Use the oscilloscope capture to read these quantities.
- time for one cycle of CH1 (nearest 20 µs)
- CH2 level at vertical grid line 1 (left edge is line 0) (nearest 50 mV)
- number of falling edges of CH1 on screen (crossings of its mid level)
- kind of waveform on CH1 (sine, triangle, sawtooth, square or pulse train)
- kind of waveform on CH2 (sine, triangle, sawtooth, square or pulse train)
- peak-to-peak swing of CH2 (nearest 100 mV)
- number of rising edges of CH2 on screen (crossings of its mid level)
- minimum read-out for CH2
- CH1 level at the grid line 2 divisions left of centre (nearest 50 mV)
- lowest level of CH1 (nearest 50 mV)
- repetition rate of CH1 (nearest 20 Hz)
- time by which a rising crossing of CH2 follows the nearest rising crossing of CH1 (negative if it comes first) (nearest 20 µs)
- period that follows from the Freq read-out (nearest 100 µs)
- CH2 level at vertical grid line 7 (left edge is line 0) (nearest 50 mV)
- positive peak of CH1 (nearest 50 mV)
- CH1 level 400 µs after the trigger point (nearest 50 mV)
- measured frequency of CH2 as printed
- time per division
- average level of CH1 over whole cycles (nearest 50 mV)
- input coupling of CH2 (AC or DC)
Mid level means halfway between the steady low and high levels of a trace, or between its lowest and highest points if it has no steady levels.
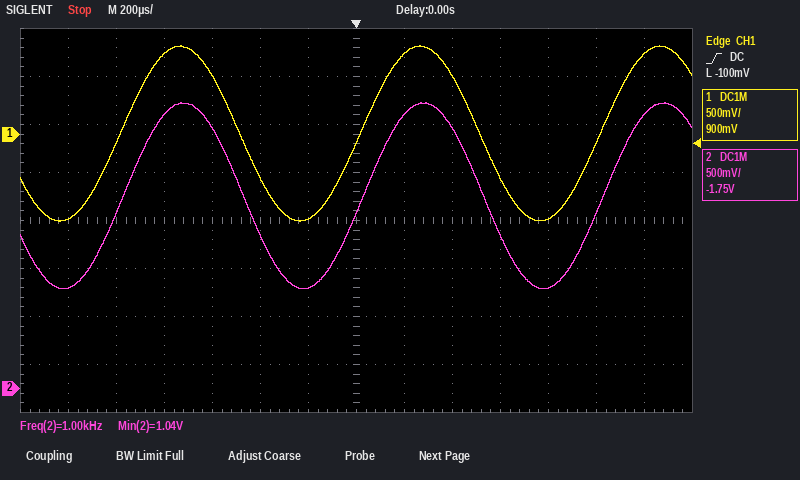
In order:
1.00 ms
1.05 V
2
sine
sine
1.90 V
3
1.04 V
-450 mV
-900 mV
1.00 kHz
+20 µs
1.0 ms
1.80 V
900 mV
600 mV
1.00 kHz
200 µs
0 mV
DC
